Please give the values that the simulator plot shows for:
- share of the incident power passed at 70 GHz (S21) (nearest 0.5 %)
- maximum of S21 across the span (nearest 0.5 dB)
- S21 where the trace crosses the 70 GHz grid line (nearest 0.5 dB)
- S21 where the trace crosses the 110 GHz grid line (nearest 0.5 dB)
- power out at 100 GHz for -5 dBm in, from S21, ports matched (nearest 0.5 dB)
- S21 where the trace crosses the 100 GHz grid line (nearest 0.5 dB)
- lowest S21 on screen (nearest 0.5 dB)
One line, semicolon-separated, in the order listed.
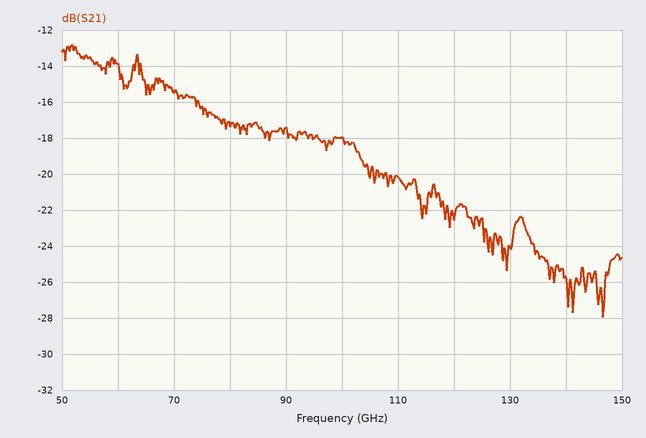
3.0 %; -13.0 dB; -15.5 dB; -20.0 dB; -23.0 dBm; -18.0 dB; -28.0 dB
